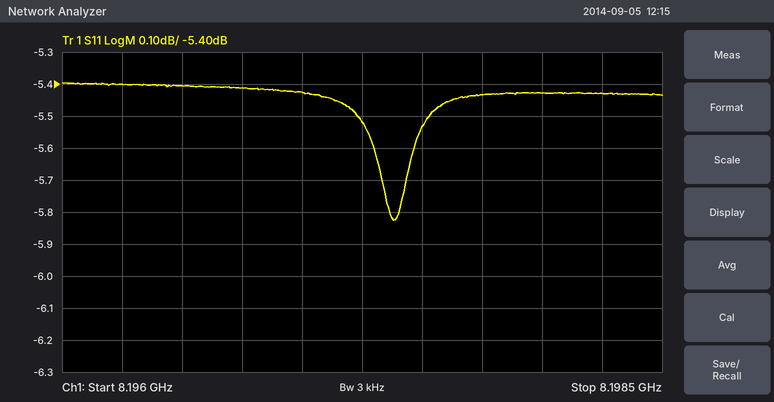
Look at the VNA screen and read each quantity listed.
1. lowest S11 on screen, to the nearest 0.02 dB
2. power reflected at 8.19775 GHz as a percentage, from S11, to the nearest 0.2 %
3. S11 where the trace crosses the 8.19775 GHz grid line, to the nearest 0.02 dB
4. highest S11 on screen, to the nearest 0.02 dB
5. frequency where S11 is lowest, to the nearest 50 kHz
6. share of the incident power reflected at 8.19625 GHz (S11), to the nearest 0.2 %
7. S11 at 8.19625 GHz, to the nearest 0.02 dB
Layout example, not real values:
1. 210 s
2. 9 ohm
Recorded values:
1. -5.82 dB
2. 28.6 %
3. -5.44 dB
4. -5.40 dB
5. 8.19740 GHz
6. 28.8 %
7. -5.40 dB
